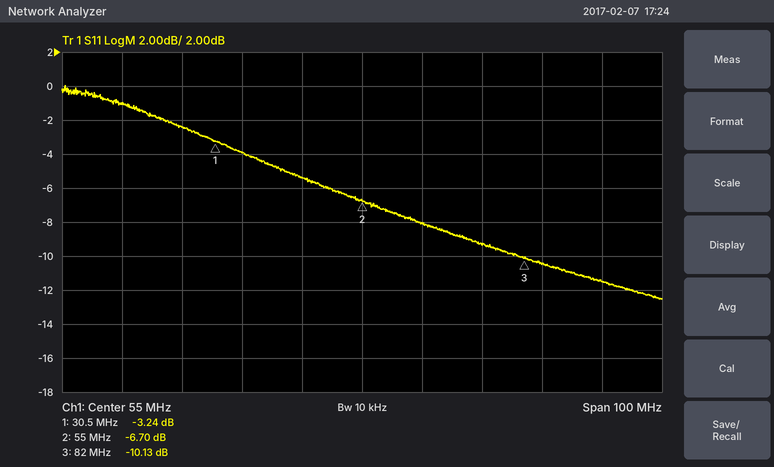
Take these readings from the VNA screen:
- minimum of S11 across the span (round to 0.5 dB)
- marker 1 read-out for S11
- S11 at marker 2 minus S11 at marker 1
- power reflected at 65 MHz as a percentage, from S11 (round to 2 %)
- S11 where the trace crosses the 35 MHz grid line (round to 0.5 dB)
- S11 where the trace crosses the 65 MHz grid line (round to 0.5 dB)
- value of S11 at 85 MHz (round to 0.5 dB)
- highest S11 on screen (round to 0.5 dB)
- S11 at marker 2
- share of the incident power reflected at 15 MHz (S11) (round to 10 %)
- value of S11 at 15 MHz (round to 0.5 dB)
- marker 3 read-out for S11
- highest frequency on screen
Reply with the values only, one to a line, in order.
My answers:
-12.5 dB
-3.24 dB
-3.46 dB
16 %
-4.0 dB
-8.0 dB
-10.5 dB
0.0 dB
-6.70 dB
80 %
-1.0 dB
-10.13 dB
105 MHz
